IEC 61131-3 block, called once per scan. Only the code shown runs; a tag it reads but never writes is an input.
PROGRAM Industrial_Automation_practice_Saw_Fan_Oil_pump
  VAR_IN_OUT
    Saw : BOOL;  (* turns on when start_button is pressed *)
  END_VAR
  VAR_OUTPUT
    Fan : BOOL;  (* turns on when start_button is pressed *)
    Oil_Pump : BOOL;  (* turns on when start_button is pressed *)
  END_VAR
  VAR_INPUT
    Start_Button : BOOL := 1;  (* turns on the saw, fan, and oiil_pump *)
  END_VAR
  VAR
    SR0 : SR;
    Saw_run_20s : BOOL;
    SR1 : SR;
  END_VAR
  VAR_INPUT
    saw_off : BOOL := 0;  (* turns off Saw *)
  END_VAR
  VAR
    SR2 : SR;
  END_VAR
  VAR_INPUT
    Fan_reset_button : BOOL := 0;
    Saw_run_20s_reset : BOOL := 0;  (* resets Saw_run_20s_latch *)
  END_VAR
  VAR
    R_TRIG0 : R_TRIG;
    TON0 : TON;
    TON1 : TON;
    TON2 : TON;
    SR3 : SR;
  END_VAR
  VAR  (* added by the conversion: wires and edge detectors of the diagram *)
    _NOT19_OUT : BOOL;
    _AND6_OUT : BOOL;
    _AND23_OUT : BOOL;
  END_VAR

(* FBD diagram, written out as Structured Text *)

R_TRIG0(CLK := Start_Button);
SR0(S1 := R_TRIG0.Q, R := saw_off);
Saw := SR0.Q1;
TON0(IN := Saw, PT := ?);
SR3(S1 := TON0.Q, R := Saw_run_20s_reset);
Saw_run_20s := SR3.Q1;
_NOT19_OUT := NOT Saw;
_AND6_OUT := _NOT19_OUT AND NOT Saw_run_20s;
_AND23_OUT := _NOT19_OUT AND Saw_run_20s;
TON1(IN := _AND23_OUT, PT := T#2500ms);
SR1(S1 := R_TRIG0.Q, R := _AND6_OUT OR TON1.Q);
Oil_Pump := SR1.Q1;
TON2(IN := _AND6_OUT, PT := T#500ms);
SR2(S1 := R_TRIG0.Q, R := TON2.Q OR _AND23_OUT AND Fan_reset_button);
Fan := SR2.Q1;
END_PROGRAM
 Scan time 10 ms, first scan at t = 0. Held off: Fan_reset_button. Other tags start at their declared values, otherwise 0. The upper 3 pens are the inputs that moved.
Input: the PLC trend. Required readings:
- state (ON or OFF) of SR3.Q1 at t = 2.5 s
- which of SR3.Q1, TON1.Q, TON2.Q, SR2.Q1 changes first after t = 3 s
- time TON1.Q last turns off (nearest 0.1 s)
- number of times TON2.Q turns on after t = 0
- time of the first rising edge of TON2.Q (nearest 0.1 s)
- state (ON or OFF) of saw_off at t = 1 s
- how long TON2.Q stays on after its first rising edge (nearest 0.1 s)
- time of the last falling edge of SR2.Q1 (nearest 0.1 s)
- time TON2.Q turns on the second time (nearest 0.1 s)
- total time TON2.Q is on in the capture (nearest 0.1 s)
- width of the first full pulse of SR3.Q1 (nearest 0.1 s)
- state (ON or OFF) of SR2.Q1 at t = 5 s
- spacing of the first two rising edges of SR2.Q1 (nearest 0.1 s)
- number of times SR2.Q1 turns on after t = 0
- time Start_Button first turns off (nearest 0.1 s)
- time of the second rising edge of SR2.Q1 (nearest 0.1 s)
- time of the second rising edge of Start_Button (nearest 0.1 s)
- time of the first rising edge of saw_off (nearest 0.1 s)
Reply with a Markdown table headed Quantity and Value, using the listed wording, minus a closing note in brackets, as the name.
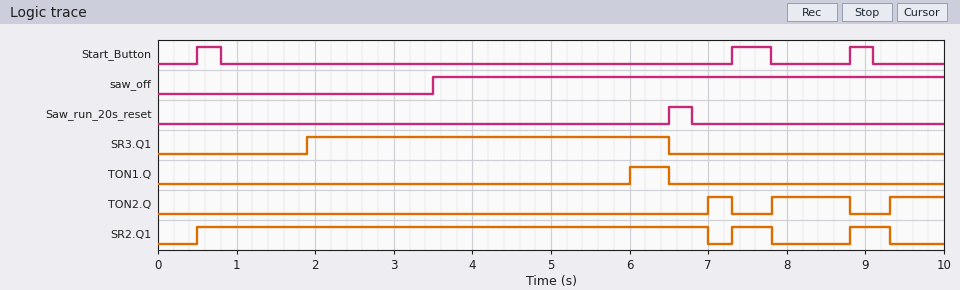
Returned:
| Quantity | Value |
|---|---|
| state (ON or OFF) of SR3.Q1 at t = 2.5 s | ON |
| which of SR3.Q1, TON1.Q, TON2.Q, SR2.Q1 changes first after t = 3 s | TON1.Q |
| time TON1.Q last turns off | 6.5 s |
| number of times TON2.Q turns on after t = 0 | 3 |
| time of the first rising edge of TON2.Q | 7.0 s |
| state (ON or OFF) of saw_off at t = 1 s | OFF |
| how long TON2.Q stays on after its first rising edge | 0.3 s |
| time of the last falling edge of SR2.Q1 | 9.3 s |
| time TON2.Q turns on the second time | 7.8 s |
| total time TON2.Q is on in the capture | 2.0 s |
| width of the first full pulse of SR3.Q1 | 4.6 s |
| state (ON or OFF) of SR2.Q1 at t = 5 s | ON |
| spacing of the first two rising edges of SR2.Q1 | 6.8 s |
| number of times SR2.Q1 turns on after t = 0 | 3 |
| time Start_Button first turns off | 0.8 s |
| time of the second rising edge of SR2.Q1 | 7.3 s |
| time of the second rising edge of Start_Button | 7.3 s |
| time of the first rising edge of saw_off | 3.5 s |
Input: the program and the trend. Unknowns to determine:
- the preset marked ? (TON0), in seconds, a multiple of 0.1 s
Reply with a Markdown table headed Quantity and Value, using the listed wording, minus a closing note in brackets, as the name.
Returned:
| Quantity | Value |
|---|---|
| the preset marked ? (TON0), in seconds, a multiple of 0.1 s | 1.4 s |
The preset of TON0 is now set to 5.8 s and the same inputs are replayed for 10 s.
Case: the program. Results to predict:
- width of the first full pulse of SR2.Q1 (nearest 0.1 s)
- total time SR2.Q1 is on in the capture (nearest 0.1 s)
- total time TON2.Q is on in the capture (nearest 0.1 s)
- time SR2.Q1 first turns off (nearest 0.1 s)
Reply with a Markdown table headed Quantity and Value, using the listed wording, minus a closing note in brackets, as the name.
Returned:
| Quantity | Value |
|---|---|
| width of the first full pulse of SR2.Q1 | 3.5 s |
| total time SR2.Q1 is on in the capture | 4.5 s |
| total time TON2.Q is on in the capture | 5.0 s |
| time SR2.Q1 first turns off | 4.0 s |
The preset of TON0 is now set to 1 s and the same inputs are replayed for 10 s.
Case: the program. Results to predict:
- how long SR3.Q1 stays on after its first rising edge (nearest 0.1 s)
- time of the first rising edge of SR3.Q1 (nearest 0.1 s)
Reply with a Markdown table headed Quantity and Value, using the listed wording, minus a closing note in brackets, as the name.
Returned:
| Quantity | Value |
|---|---|
| how long SR3.Q1 stays on after its first rising edge | 5.0 s |
| time of the first rising edge of SR3.Q1 | 1.5 s |
